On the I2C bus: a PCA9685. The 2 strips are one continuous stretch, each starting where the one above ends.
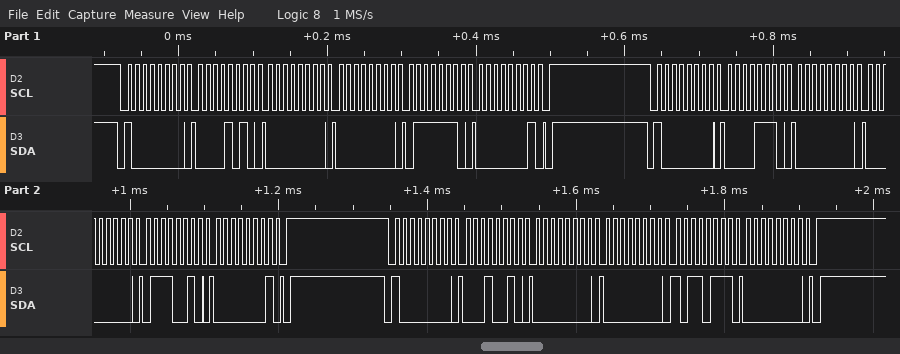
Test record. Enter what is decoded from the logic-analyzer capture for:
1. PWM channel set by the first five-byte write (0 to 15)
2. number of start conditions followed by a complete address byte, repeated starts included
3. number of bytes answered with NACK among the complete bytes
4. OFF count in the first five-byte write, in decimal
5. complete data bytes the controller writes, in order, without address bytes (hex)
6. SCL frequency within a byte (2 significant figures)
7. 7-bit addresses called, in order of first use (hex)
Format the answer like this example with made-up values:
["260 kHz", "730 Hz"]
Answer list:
["1", "3", "0", "382", "0A 00 00 7E 01 0E 00 00 72 01 12 00 00 B7 00", "100 kHz", "0x40"]
